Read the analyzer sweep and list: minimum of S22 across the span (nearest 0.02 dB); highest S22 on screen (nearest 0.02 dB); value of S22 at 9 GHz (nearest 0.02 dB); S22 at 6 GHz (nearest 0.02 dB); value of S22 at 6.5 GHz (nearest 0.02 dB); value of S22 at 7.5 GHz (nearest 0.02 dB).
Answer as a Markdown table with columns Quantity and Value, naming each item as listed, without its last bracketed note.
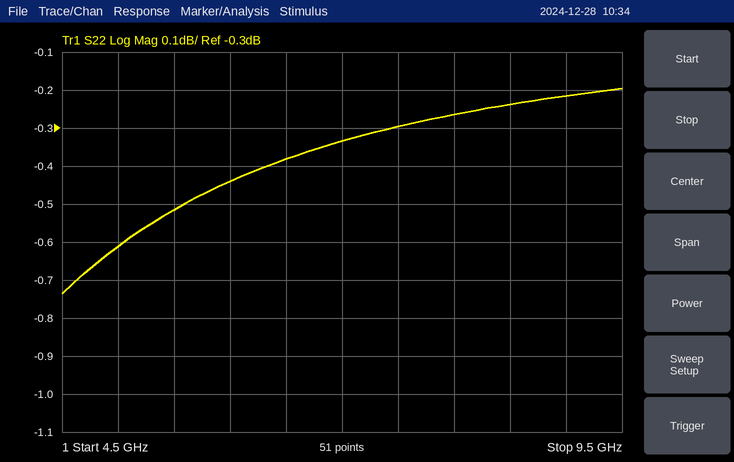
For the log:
| Quantity | Value |
|---|---|
| minimum of S22 across the span | -0.74 dB |
| highest S22 on screen | -0.20 dB |
| value of S22 at 9 GHz | -0.22 dB |
| S22 at 6 GHz | -0.44 dB |
| value of S22 at 6.5 GHz | -0.38 dB |
| value of S22 at 7.5 GHz | -0.30 dB |
